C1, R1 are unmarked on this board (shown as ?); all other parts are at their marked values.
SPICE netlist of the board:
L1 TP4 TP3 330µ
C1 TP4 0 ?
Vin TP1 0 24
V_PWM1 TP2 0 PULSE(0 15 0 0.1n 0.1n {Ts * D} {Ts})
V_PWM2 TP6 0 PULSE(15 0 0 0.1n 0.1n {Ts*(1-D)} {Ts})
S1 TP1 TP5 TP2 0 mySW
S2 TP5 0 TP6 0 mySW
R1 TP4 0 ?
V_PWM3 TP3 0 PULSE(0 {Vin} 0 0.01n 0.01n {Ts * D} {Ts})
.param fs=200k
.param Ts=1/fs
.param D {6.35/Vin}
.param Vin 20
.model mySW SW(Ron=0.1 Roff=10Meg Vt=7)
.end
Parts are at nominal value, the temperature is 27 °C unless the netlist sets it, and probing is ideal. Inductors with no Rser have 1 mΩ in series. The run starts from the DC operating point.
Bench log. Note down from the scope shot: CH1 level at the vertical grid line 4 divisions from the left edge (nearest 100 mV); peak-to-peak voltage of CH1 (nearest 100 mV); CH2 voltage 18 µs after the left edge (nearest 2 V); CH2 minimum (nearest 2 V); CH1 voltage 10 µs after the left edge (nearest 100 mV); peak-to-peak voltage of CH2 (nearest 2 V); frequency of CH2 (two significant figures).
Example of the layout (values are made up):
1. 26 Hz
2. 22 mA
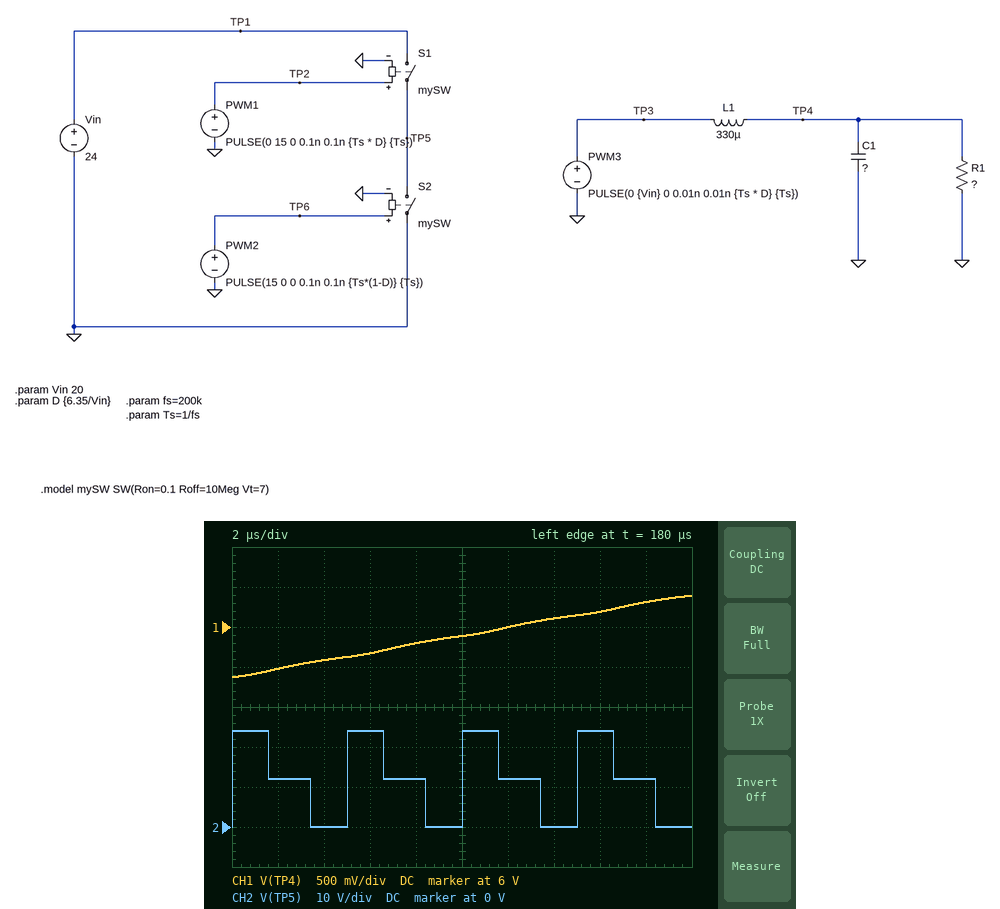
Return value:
1. 5.8 V
2. 1.0 V
3. 12 V
4. 0 V
5. 5.9 V
6. 24 V
7. 200 kHz
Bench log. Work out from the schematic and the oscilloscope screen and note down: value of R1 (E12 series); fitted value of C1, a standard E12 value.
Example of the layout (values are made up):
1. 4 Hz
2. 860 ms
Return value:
1. 33 Ω
2. 1.8 µF
